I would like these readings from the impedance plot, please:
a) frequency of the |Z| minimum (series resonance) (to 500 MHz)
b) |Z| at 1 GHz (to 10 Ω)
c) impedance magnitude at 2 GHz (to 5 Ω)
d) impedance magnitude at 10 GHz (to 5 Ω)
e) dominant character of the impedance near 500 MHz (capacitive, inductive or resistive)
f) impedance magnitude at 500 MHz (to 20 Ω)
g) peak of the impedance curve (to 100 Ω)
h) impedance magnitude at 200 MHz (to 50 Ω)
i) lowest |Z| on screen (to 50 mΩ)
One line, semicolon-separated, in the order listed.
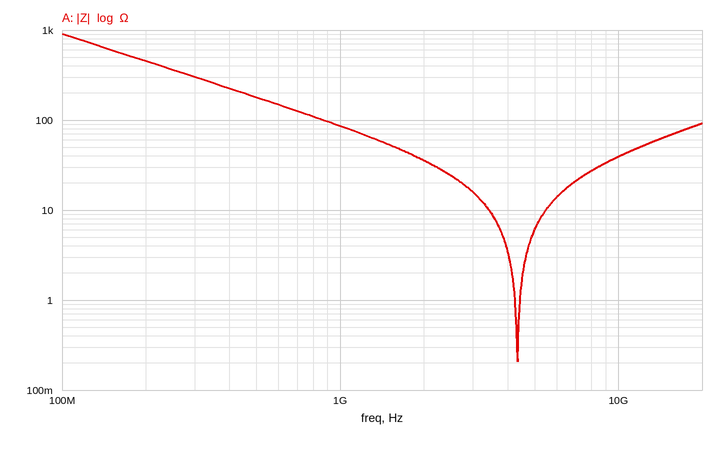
4.5 GHz; 90 Ω; 35 Ω; 40 Ω; capacitive; 180 Ω; 900 Ω; 450 Ω; 200 mΩ
